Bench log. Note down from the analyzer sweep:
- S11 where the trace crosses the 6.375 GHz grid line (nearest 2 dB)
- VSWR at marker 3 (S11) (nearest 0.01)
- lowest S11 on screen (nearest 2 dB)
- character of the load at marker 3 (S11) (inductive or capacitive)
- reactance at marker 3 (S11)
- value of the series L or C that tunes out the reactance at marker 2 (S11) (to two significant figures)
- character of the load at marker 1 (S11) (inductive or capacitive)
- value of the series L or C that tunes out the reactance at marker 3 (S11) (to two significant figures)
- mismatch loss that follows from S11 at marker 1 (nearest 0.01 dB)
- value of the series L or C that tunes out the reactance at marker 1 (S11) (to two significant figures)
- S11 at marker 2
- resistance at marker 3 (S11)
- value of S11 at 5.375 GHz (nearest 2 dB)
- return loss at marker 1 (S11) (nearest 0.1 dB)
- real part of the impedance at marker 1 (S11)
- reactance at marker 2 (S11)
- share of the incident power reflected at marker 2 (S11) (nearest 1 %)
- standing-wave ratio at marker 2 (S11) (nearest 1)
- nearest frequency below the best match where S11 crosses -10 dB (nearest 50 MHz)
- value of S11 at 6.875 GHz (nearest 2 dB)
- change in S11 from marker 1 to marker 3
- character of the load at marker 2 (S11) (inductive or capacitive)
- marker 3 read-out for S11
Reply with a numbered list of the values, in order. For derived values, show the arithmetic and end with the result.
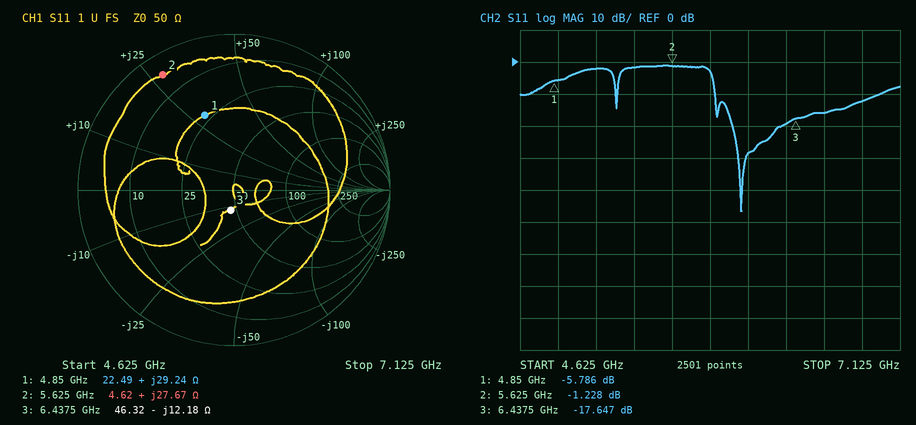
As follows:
1. -20 dB
2. (1 + 0.1311)/(1 − 0.1311) ≈ 1.30
3. -46 dB
4. capacitive
5. -12.18 Ω
6. C = 1/(2π × 5.625 GHz × 27.67 Ω) ≈ 1.0 pF
7. inductive
8. L = 12.18 Ω/(2π × 6.4375 GHz) ≈ 301 pH, so 300 pH to two significant figures
9. −10 log10(1 − 10^(-5.786/10)) ≈ 1.33 dB
10. C = 1/(2π × 4.85 GHz × 29.24 Ω) ≈ 1.1 pF
11. -1.228 dB
12. 46.32 Ω
13. -2 dB
14. 5.8 dB
15. 22.49 Ω
16. +27.67 Ω
17. 10^(-1.228/10) ≈ 75 %
18. 14
19. 5.90 GHz
20. -12 dB
21. -17.647 − (-5.786) = -11.861 dB
22. inductive
23. -17.647 dB
